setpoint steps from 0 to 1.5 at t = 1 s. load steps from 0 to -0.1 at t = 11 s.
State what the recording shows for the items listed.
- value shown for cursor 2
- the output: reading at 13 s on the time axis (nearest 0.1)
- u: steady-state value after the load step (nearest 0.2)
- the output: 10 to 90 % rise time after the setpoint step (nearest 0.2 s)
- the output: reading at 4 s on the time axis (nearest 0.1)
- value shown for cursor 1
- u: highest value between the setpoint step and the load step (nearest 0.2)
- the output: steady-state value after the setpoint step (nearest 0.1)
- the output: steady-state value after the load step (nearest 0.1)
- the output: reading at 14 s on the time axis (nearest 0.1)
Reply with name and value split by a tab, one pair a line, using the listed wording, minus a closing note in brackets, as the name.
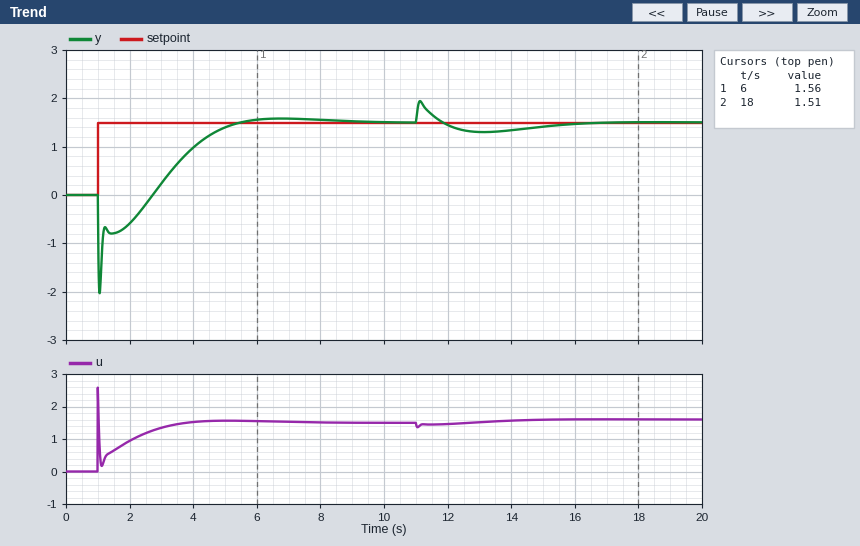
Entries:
value shown for cursor 2	1.51
the output: reading at 13 s on the time axis	1.3
u: steady-state value after the load step	1.6
the output: 10 to 90 % rise time after the setpoint step	2.0 s
the output: reading at 4 s on the time axis	1.0
value shown for cursor 1	1.56
u: highest value between the setpoint step and the load step	2.6
the output: steady-state value after the setpoint step	1.5
the output: steady-state value after the load step	1.5
the output: reading at 14 s on the time axis	1.3
